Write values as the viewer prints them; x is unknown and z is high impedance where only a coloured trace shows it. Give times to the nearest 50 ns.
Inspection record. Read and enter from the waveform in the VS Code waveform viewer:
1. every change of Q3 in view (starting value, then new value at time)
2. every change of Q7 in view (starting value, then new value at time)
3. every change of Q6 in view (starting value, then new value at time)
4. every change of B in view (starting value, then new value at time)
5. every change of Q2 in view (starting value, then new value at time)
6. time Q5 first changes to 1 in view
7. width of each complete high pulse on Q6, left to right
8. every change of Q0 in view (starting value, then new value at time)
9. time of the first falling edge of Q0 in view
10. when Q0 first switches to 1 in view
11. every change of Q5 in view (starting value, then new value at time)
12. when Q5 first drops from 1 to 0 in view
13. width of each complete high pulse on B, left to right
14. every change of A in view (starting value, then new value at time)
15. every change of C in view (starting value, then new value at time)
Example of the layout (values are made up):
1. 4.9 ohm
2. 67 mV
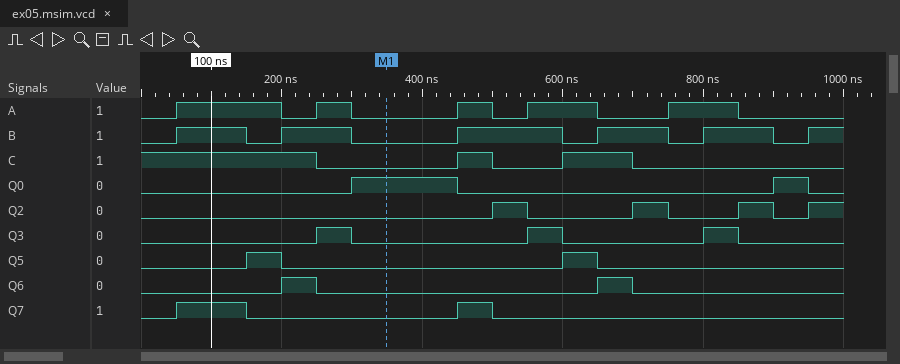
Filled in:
1. 0, 1 at 250 ns, 0 at 300 ns, 1 at 550 ns, 0 at 600 ns, 1 at 800 ns, 0 at 850 ns
2. 0, 1 at 50 ns, 0 at 150 ns, 1 at 450 ns, 0 at 500 ns
3. 0, 1 at 200 ns, 0 at 250 ns, 1 at 650 ns, 0 at 700 ns
4. 0, 1 at 50 ns, 0 at 150 ns, 1 at 200 ns, 0 at 300 ns, 1 at 450 ns, 0 at 600 ns, 1 at 650 ns, 0 at 750 ns, 1 at 800 ns, 0 at 900 ns, 1 at 950 ns
5. 0, 1 at 500 ns, 0 at 550 ns, 1 at 700 ns, 0 at 750 ns, 1 at 850 ns, 0 at 900 ns, 1 at 950 ns
6. 150 ns
7. 50 ns, 50 ns
8. 0, 1 at 300 ns, 0 at 450 ns, 1 at 900 ns, 0 at 950 ns
9. 450 ns
10. 300 ns
11. 0, 1 at 150 ns, 0 at 200 ns, 1 at 600 ns, 0 at 650 ns
12. 200 ns
13. 100 ns, 100 ns, 150 ns, 100 ns, 100 ns
14. 0, 1 at 50 ns, 0 at 200 ns, 1 at 250 ns, 0 at 300 ns, 1 at 450 ns, 0 at 500 ns, 1 at 550 ns, 0 at 650 ns, 1 at 750 ns, 0 at 850 ns
15. 1, 0 at 250 ns, 1 at 450 ns, 0 at 500 ns, 1 at 600 ns, 0 at 700 ns
